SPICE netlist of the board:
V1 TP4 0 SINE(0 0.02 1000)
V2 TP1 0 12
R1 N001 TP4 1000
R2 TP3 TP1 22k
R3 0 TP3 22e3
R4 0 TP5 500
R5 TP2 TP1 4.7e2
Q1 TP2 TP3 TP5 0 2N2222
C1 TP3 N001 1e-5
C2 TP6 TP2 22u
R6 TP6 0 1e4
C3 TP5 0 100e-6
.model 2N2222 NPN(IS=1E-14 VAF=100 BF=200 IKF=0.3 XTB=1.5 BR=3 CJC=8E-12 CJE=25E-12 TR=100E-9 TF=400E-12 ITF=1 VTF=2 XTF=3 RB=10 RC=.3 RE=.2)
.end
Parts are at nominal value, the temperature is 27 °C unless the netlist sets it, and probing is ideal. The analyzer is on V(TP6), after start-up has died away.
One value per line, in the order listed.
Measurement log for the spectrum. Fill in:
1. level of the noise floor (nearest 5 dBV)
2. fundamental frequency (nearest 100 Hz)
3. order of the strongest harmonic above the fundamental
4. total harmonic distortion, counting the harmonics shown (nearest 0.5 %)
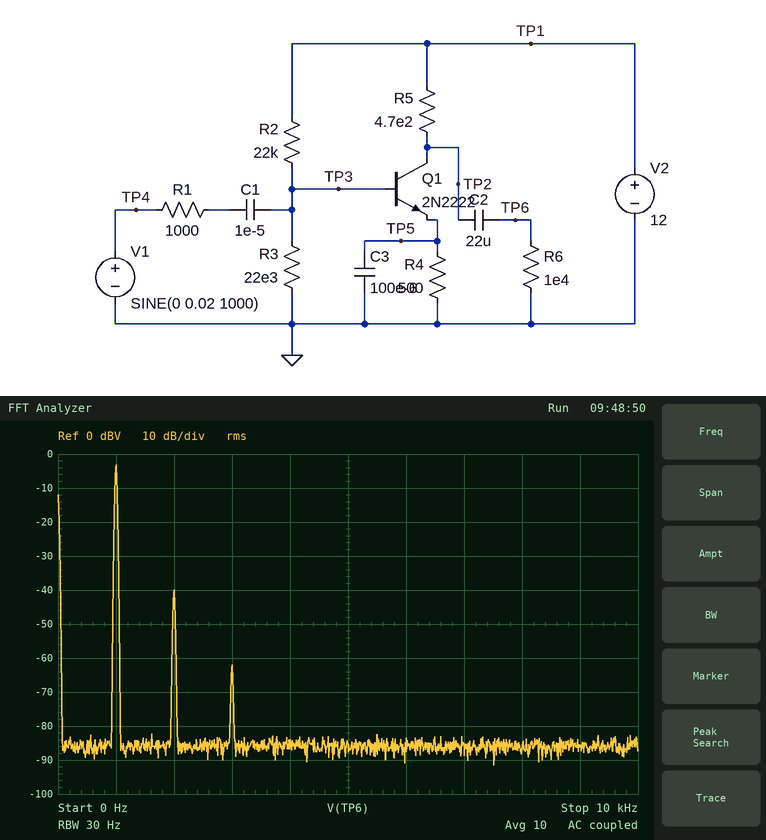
-85 dBV
1.0 kHz
2
1.5 %
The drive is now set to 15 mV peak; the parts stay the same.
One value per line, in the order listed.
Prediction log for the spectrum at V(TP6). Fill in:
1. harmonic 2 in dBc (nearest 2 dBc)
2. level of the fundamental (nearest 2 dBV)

-40 dBc
-6 dBV
